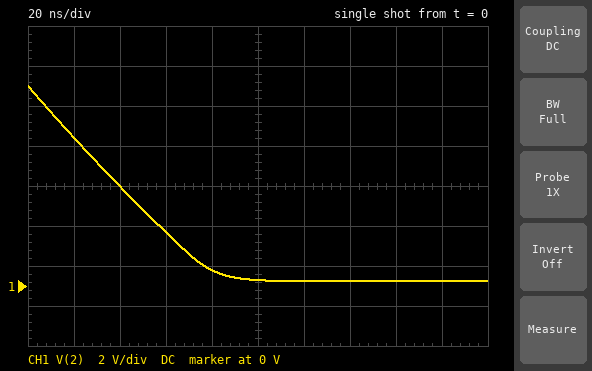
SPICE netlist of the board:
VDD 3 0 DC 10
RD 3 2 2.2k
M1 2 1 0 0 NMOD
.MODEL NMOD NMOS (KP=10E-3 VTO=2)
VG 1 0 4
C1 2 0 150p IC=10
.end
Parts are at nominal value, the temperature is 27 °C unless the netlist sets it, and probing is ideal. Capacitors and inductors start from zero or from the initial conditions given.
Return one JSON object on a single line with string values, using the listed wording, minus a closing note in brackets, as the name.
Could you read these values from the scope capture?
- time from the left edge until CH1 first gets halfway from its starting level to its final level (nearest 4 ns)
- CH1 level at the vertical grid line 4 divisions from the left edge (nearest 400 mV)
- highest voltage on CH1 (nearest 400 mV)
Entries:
{"time from the left edge until CH1 first gets halfway from its starting level to its final level": "40 ns", "CH1 level at the vertical grid line 4 divisions from the left edge": "800 mV", "highest voltage on CH1": "10.0 V"}
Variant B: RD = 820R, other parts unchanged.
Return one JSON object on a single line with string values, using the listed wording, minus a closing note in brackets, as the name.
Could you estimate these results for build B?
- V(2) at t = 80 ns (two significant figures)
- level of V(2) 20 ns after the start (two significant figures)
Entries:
{"V(2) at t = 80 ns": "2.2 V", "level of V(2) 20 ns after the start": "7.5 V"}
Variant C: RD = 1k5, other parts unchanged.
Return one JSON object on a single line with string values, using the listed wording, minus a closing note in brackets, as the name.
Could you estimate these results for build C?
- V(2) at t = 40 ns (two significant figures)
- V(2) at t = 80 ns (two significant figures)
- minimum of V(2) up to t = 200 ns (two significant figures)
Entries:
{"V(2) at t = 40 ns": "5.1 V", "V(2) at t = 80 ns": "1.1 V", "minimum of V(2) up to t = 200 ns": "350 mV"}
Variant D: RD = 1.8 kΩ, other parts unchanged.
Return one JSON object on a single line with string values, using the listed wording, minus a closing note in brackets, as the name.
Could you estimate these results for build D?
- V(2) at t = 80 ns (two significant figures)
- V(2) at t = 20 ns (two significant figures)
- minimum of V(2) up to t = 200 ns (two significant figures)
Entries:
{"V(2) at t = 80 ns": "940 mV", "V(2) at t = 20 ns": "7.4 V", "minimum of V(2) up to t = 200 ns": "290 mV"}
